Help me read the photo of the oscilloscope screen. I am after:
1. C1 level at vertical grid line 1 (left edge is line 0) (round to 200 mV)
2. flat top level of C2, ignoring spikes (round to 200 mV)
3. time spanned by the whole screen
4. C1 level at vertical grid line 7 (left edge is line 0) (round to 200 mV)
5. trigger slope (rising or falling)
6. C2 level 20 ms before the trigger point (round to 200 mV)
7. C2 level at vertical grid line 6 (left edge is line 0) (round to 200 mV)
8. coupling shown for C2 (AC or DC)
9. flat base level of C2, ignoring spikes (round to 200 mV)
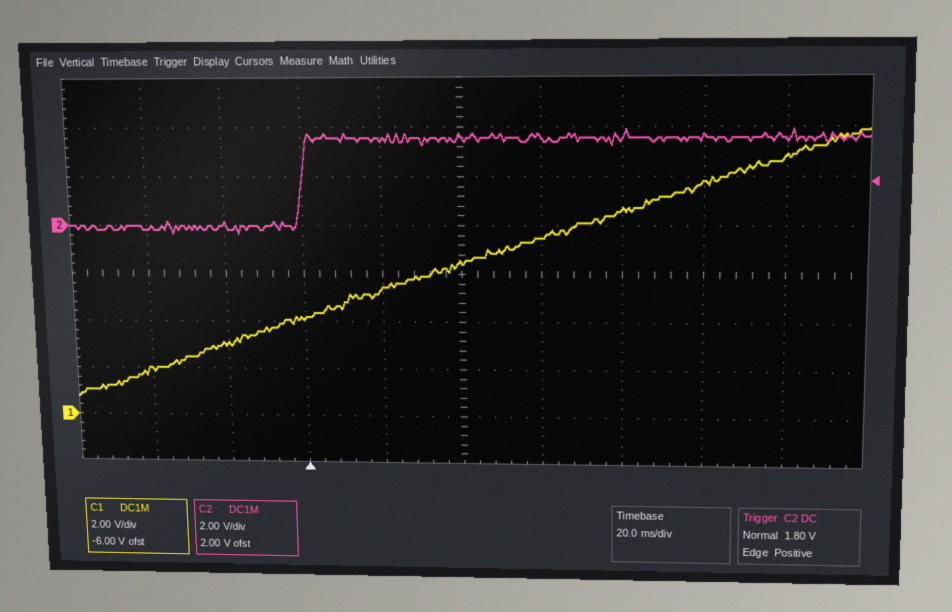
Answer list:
2.0 V
3.6 V
200 ms
8.6 V
rising
0.0 V
3.6 V
DC
0.0 V
